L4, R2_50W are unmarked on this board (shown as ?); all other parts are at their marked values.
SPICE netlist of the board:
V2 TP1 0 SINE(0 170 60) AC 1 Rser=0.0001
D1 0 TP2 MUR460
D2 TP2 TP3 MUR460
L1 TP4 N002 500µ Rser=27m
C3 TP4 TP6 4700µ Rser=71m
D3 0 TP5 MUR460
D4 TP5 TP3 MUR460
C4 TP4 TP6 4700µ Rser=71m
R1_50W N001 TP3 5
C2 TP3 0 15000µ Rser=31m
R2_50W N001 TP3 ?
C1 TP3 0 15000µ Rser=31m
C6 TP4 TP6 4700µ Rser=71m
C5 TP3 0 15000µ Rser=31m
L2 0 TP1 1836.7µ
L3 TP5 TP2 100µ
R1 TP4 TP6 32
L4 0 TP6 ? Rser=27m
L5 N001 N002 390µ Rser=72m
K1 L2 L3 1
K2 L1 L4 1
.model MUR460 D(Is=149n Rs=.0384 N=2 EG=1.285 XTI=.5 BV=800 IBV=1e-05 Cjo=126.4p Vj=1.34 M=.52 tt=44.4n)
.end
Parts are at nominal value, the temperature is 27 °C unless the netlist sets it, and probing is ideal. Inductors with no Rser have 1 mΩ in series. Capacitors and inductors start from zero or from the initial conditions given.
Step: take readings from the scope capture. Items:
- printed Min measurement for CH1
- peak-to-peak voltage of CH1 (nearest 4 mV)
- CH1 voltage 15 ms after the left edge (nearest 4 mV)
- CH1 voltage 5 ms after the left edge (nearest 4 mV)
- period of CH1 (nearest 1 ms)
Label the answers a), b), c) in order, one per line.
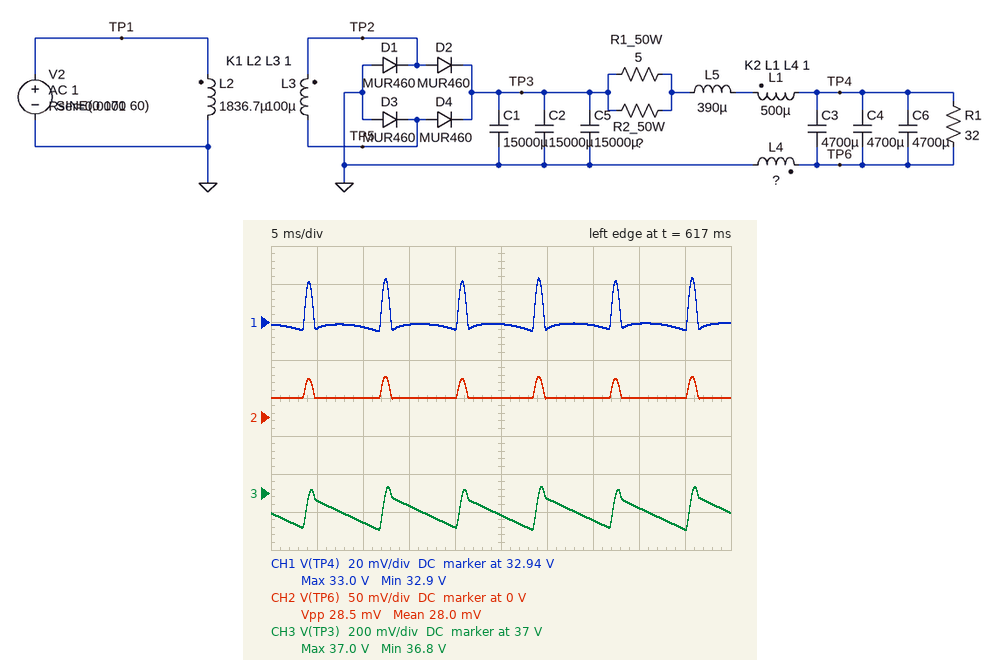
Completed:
a) 32.9 V
b) 28 mV
c) 32.940 V
d) 32.936 V
e) 8 ms
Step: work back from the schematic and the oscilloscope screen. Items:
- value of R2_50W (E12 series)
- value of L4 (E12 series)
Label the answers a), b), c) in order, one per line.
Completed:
a) 15 Ω
b) 150 µH
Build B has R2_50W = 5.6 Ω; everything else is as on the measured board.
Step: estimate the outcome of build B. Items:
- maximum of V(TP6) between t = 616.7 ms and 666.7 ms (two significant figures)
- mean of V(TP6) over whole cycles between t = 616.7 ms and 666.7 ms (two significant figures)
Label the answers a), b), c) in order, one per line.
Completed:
a) 59 mV
b) 29 mV
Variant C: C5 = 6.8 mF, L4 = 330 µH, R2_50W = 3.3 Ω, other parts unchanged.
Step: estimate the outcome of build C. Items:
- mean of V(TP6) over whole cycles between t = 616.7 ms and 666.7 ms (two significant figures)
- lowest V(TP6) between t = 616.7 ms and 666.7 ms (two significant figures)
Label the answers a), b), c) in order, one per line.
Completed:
a) 29 mV
b) 19 mV
